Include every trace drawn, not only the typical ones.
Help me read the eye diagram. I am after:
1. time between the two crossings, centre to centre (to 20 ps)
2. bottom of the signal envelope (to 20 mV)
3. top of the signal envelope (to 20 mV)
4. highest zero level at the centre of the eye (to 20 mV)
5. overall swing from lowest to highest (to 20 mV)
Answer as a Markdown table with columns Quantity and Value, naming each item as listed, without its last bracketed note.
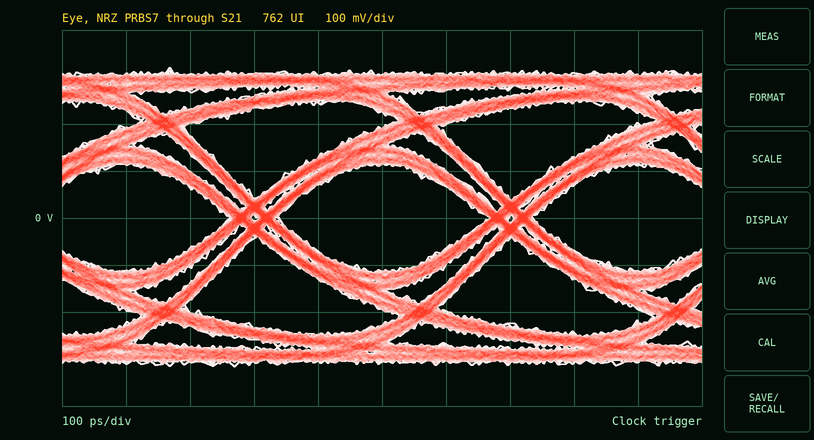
| Quantity | Value |
|---|---|
| time between the two crossings, centre to centre | 400 ps |
| bottom of the signal envelope | -320 mV |
| top of the signal envelope | 320 mV |
| highest zero level at the centre of the eye | -120 mV |
| overall swing from lowest to highest | 640 mV |
